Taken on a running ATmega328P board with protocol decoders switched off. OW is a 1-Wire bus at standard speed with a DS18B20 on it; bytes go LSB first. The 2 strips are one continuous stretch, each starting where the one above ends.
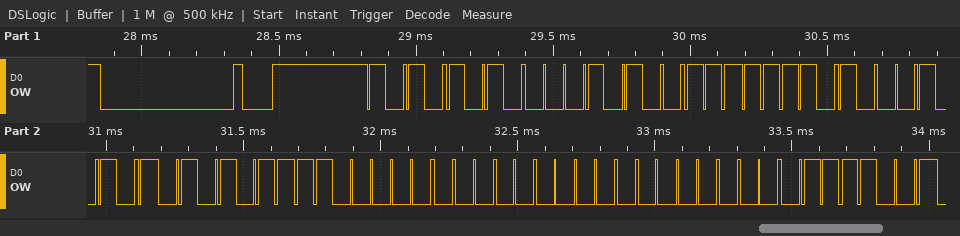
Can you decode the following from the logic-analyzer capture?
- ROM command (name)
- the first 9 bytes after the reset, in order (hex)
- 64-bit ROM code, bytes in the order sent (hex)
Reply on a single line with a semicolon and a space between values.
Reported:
Match ROM; 55 28 7F 51 D5 03 00 00 9E; 28 7F 51 D5 03 00 00 9E
